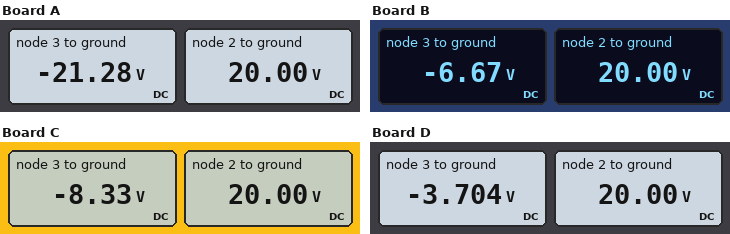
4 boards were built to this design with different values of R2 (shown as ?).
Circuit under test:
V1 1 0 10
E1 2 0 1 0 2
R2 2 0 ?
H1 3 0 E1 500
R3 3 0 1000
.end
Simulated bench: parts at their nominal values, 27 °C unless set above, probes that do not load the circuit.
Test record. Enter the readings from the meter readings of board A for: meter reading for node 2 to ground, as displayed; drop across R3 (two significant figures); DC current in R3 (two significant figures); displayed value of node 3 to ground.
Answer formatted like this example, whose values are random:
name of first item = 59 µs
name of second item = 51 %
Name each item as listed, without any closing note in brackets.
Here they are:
meter reading for node 2 to ground, as displayed = 20.00 V
drop across R3 = 21 V
DC current in R3 = 21 mA
displayed value of node 3 to ground = -21.28 V
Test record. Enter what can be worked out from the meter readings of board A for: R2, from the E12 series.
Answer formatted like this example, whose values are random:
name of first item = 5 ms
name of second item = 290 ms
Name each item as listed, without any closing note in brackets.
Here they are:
R2, from the E12 series = 470 Ω
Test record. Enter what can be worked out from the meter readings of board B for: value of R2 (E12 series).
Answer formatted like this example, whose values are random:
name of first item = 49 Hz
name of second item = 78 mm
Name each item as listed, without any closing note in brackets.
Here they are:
value of R2 = 1.5 kΩ
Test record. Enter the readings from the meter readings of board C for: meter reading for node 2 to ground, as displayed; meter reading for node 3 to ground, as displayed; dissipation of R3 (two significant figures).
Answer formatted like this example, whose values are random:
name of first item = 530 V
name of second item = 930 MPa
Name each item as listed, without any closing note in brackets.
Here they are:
meter reading for node 2 to ground, as displayed = 20.00 V
meter reading for node 3 to ground, as displayed = -8.33 V
dissipation of R3 = 69 mW
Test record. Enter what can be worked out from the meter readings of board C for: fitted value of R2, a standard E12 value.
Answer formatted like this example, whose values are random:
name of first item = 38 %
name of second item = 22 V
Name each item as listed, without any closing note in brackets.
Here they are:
fitted value of R2, a standard E12 value = 1.2 kΩ
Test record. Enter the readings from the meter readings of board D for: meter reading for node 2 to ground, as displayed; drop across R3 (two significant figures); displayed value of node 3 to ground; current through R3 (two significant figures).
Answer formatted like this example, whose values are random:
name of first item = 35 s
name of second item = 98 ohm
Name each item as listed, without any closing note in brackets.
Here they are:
meter reading for node 2 to ground, as displayed = 20.00 V
drop across R3 = 3.7 V
displayed value of node 3 to ground = -3.704 V
current through R3 = 3.7 mA
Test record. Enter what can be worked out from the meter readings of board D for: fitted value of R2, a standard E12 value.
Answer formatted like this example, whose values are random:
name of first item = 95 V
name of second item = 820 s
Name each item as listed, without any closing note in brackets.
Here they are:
fitted value of R2, a standard E12 value = 2.7 kΩ
